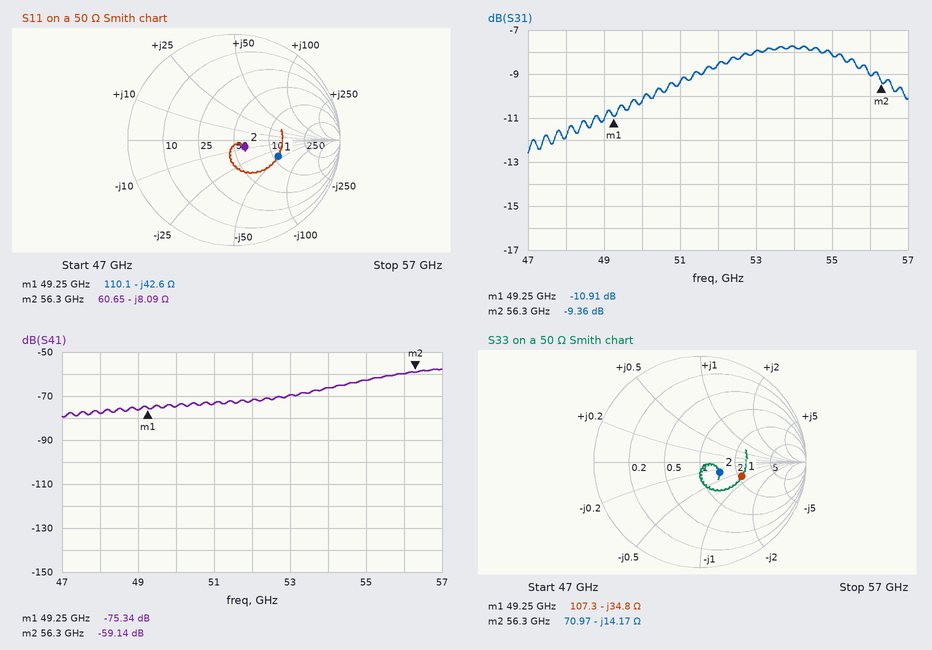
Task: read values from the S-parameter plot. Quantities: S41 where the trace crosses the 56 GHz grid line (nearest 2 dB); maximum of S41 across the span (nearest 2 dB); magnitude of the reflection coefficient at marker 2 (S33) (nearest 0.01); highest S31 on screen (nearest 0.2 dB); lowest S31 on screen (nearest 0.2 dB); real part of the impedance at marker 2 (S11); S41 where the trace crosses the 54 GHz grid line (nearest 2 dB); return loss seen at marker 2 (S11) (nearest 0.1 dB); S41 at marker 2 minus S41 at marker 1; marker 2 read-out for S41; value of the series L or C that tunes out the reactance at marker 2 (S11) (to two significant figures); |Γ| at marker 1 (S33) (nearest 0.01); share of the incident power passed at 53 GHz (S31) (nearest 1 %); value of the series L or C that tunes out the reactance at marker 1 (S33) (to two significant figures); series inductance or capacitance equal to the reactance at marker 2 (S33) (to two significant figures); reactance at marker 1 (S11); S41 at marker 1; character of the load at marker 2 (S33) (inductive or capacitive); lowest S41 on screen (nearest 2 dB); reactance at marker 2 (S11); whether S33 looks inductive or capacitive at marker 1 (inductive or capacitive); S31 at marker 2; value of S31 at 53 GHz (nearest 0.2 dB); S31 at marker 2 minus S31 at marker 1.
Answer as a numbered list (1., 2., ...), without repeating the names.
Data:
1. -60 dB
2. -58 dB
3. 0.21
4. -7.8 dB
5. -12.6 dB
6. 60.65 Ω
7. -66 dB
8. 18.4 dB
9. 16.20 dB
10. -59.14 dB
11. 23 pH
12. 0.42
13. 16 %
14. 110 pH
15. 200 fF
16. -42.6 Ω
17. -75.34 dB
18. capacitive
19. -80 dB
20. -8.09 Ω
21. capacitive
22. -9.36 dB
23. -8.0 dB
24. 1.55 dB
